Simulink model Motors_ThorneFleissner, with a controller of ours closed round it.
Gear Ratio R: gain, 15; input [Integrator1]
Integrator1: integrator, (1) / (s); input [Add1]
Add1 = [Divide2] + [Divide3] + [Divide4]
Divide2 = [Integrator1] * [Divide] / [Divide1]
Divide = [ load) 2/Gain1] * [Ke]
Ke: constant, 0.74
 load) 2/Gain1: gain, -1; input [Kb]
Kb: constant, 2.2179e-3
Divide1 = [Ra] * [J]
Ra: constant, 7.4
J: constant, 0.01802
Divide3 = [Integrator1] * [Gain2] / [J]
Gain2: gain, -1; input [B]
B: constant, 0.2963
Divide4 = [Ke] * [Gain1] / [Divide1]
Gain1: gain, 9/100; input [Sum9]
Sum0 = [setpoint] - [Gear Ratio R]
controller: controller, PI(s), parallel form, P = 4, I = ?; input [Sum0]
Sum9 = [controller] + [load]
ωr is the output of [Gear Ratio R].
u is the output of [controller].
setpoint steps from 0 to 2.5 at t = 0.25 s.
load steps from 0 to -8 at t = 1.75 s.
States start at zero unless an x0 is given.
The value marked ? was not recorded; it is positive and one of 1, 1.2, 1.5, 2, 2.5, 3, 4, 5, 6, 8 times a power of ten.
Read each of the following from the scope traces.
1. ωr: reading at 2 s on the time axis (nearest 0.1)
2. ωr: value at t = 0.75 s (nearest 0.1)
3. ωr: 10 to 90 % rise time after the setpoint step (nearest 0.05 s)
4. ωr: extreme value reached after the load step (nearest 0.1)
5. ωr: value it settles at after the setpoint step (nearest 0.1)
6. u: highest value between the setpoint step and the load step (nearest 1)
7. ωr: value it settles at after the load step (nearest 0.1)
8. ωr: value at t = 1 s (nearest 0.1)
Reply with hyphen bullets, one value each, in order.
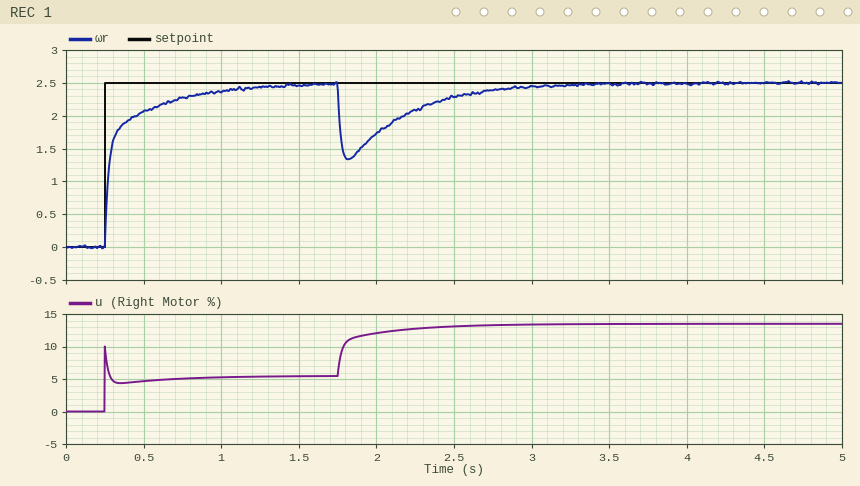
- 1.7
- 2.3
- 0.45 s
- 1.3
- 2.5
- 10
- 2.5
- 2.4
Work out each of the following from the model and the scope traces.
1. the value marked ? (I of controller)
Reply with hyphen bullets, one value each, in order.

- 15
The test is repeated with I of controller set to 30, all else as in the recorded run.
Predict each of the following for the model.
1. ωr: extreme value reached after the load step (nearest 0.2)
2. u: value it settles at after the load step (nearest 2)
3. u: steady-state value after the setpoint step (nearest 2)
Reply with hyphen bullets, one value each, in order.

- 1.4
- 14
- 6
